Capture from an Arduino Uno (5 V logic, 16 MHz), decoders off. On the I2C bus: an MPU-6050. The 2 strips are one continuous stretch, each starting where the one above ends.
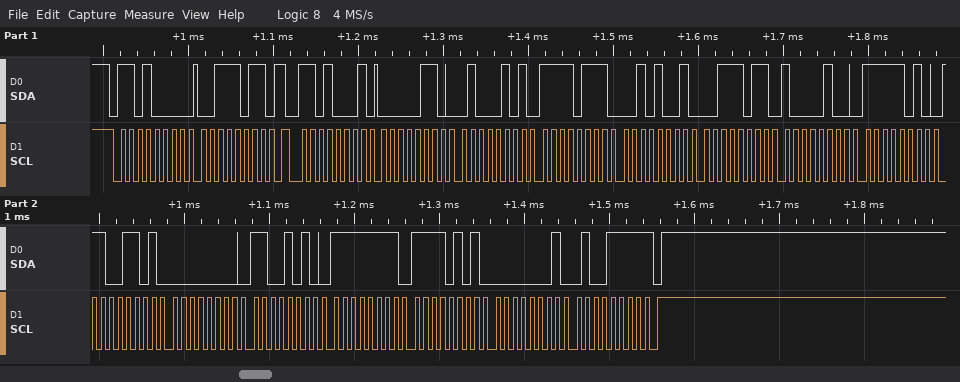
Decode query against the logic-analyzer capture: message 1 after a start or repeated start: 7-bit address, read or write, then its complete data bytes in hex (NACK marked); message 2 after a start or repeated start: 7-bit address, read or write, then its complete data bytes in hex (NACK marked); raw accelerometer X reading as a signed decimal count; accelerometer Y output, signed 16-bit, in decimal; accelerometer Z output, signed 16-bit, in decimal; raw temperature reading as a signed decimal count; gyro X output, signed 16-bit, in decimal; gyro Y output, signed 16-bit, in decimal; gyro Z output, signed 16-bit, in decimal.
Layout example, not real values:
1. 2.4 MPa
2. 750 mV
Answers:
1. 0x68 write: 3B
2. 0x68 read: 06 45 F7 29 3B 84 FA CD 00 CA FF F5 01 4F NACK
3. 1605
4. -2263
5. 15236
6. -1331
7. 202
8. -11
9. 335
